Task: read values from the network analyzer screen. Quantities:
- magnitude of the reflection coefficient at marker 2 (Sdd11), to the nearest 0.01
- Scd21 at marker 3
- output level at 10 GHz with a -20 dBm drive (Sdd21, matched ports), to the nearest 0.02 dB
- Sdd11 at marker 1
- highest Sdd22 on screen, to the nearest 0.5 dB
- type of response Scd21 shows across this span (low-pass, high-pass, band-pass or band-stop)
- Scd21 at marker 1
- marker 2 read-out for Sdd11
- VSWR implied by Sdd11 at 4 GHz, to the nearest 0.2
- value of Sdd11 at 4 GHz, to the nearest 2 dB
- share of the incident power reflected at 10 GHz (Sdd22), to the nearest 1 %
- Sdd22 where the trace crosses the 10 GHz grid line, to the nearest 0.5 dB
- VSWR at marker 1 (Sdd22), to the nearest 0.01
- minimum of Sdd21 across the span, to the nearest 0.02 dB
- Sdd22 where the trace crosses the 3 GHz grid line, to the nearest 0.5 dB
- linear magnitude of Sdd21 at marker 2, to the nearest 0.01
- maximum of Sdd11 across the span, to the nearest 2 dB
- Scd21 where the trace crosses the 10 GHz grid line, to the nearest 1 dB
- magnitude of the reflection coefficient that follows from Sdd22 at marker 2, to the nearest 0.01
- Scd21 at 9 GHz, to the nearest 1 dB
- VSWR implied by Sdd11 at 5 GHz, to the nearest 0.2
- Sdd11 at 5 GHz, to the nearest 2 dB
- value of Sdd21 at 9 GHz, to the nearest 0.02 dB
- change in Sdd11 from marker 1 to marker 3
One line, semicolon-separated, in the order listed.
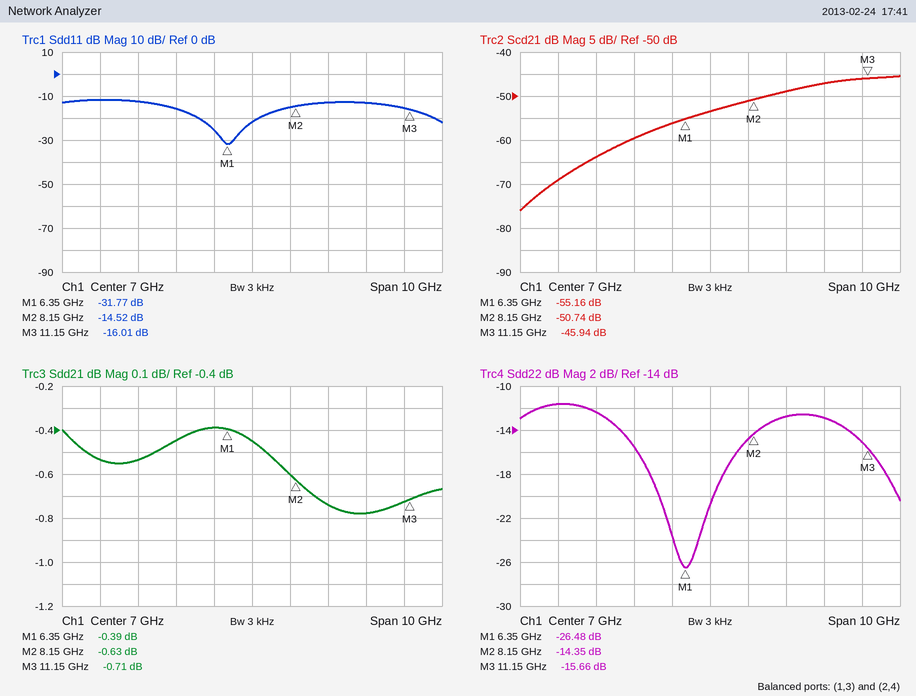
0.19; -45.94 dB; -20.78 dBm; -31.77 dB; -11.5 dB; high-pass; -55.16 dB; -14.52 dB; 1.6; -12 dB; 5 %; -13.0 dB; 1.10; -0.78 dB; -11.5 dB; 0.93; -12 dB; -47 dB; 0.19; -49 dB; 1.4; -16 dB; -0.74 dB; 15.76 dB
